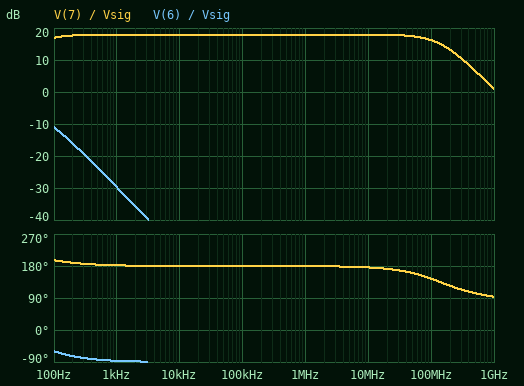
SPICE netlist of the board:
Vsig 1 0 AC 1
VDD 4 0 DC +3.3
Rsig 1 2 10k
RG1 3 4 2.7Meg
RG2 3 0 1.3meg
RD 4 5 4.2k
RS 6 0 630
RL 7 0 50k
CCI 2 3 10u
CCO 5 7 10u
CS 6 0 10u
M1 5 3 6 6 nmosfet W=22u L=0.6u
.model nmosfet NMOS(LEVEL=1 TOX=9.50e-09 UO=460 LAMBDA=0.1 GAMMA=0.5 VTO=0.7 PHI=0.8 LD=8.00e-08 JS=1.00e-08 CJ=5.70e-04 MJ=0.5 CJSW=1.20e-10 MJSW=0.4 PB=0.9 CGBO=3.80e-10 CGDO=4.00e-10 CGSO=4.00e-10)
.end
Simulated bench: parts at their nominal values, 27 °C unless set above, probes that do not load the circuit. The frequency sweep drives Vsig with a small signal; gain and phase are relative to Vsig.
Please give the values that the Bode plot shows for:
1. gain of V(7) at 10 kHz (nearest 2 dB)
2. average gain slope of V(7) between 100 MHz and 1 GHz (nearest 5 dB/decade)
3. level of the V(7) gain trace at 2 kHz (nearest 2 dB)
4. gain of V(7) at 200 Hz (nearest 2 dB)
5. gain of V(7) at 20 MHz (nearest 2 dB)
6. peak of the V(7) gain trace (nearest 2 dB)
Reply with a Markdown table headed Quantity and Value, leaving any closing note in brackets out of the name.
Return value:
| Quantity | Value |
|---|---|
| gain of V(7) at 10 kHz | 18 dB |
| average gain slope of V(7) between 100 MHz and 1 GHz | -15 dB/decade |
| level of the V(7) gain trace at 2 kHz | 18 dB |
| gain of V(7) at 200 Hz | 18 dB |
| gain of V(7) at 20 MHz | 18 dB |
| peak of the V(7) gain trace | 18 dB |
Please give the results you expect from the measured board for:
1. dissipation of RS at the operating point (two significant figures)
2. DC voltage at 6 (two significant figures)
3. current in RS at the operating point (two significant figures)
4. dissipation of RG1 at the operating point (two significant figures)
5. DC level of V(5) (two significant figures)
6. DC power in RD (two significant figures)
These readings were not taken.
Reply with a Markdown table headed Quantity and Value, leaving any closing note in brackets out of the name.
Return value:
| Quantity | Value |
|---|---|
| dissipation of RS at the operating point | 37 µW |
| DC voltage at 6 | 150 mV |
| current in RS at the operating point | 240 µA |
| dissipation of RG1 at the operating point | 1.8 µW |
| DC level of V(5) | 2.3 V |
| DC power in RD | 250 µW |
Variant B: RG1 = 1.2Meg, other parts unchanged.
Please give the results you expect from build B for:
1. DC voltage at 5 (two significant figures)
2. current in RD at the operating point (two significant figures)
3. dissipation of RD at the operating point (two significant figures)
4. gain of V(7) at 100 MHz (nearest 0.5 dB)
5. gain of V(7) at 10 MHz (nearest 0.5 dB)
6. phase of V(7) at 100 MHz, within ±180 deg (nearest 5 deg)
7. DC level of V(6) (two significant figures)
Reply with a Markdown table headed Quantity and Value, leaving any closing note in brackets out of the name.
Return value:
| Quantity | Value |
|---|---|
| DC voltage at 5 | 560 mV |
| current in RD at the operating point | 650 µA |
| dissipation of RD at the operating point | 1.8 mW |
| gain of V(7) at 100 MHz | -11.5 dB |
| gain of V(7) at 10 MHz | -11.0 dB |
| phase of V(7) at 100 MHz, within ±180 deg | 160 deg |
| DC level of V(6) | 410 mV |
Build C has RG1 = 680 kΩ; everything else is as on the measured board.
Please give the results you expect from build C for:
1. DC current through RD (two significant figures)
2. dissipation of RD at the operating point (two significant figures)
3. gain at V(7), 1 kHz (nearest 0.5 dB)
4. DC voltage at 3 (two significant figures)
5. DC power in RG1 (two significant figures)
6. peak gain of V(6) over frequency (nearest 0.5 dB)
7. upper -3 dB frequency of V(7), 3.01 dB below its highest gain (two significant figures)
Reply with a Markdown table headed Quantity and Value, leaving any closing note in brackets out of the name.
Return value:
| Quantity | Value |
|---|---|
| DC current through RD | 670 µA |
| dissipation of RD at the operating point | 1.9 mW |
| gain at V(7), 1 kHz | -22.5 dB |
| DC voltage at 3 | 2.2 V |
| DC power in RG1 | 1.9 µW |
| peak gain of V(6) over frequency | -39.5 dB |
| upper -3 dB frequency of V(7), 3.01 dB below its highest gain | 300 MHz |
